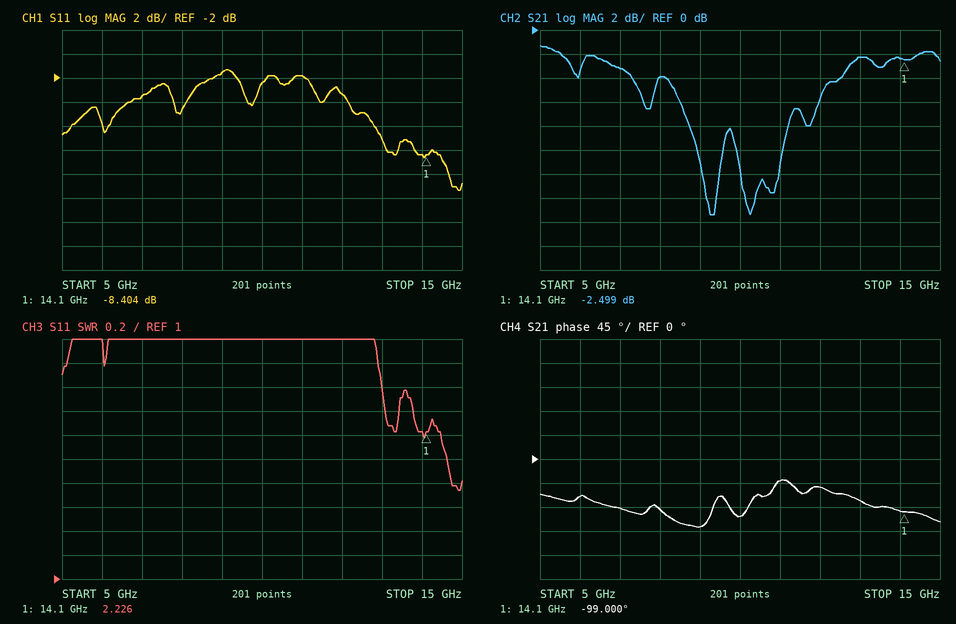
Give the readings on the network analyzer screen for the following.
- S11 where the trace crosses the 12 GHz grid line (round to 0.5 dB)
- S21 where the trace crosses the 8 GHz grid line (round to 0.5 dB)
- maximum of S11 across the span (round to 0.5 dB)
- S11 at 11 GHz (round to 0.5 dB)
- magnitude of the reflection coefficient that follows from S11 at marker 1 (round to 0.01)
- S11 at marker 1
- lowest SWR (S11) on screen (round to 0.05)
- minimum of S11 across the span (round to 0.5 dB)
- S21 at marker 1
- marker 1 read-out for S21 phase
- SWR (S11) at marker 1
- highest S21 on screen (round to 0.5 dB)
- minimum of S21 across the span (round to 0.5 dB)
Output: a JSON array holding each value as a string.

["-3.5 dB", "-4.0 dB", "-1.5 dB", "-2.0 dB", "0.38", "-8.404 dB", "1.75", "-11.5 dB", "-2.499 dB", "-99.000°", "2.226", "-1.5 dB", "-15.5 dB"]
